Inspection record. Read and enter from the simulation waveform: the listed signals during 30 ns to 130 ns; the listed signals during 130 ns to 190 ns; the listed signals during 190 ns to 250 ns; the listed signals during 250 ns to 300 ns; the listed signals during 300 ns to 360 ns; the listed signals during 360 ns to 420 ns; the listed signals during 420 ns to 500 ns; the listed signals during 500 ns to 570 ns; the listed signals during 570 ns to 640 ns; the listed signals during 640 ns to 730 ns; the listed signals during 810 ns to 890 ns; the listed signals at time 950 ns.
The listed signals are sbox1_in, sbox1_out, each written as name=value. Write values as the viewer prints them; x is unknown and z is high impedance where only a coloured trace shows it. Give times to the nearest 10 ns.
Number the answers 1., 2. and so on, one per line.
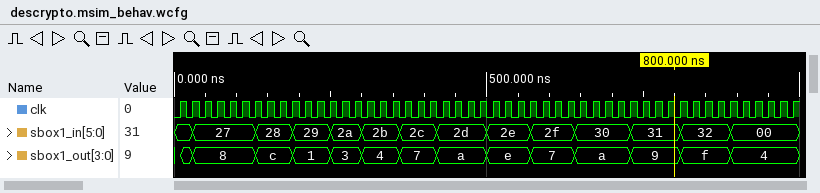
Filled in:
1. sbox1_in=27, sbox1_out=8
2. sbox1_in=28, sbox1_out=c
3. sbox1_in=29, sbox1_out=1
4. sbox1_in=2a, sbox1_out=3
5. sbox1_in=2b, sbox1_out=4
6. sbox1_in=2c, sbox1_out=7
7. sbox1_in=2d, sbox1_out=a
8. sbox1_in=2e, sbox1_out=e
9. sbox1_in=2f, sbox1_out=7
10. sbox1_in=30, sbox1_out=a
11. sbox1_in=32, sbox1_out=f
12. sbox1_in=00, sbox1_out=4
